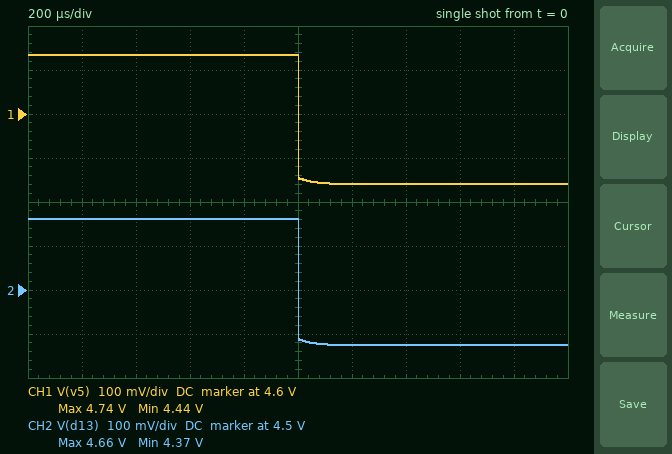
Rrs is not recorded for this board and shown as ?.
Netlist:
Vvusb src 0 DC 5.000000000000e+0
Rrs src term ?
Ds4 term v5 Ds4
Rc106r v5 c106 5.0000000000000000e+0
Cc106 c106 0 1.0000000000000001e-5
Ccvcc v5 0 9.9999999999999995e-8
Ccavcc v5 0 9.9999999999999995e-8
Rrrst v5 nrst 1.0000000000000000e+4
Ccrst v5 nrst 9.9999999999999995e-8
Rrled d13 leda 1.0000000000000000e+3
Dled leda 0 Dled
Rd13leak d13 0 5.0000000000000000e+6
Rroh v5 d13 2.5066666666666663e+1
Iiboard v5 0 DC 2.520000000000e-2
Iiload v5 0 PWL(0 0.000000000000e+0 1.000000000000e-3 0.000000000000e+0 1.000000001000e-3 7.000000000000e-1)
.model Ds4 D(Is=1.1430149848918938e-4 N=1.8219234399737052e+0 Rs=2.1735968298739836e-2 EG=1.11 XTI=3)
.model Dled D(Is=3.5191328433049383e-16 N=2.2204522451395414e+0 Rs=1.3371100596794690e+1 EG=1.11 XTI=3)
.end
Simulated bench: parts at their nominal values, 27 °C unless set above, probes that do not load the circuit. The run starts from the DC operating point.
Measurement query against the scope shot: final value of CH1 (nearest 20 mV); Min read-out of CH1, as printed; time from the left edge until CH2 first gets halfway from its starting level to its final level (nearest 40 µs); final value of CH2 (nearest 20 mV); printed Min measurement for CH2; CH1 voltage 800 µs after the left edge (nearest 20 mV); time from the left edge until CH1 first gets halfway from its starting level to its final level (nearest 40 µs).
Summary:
4.44 V
4.44 V
1.00 ms
4.38 V
4.37 V
4.74 V
1.00 ms
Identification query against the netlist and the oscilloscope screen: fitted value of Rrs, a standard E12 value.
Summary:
0.18 Ω
